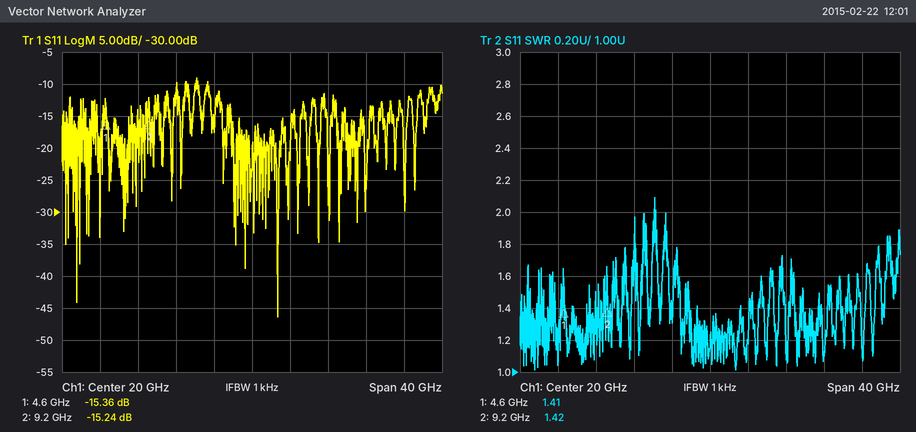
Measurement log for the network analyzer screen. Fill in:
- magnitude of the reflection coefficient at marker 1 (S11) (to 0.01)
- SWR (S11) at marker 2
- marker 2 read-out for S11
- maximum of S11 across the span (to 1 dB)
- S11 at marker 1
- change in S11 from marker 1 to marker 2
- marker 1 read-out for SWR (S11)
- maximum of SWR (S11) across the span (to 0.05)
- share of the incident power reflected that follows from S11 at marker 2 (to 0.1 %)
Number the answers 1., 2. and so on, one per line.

1. 0.17
2. 1.42
3. -15.24 dB
4. -9 dB
5. -15.36 dB
6. 0.12 dB
7. 1.41
8. 2.10
9. 3.0 %
